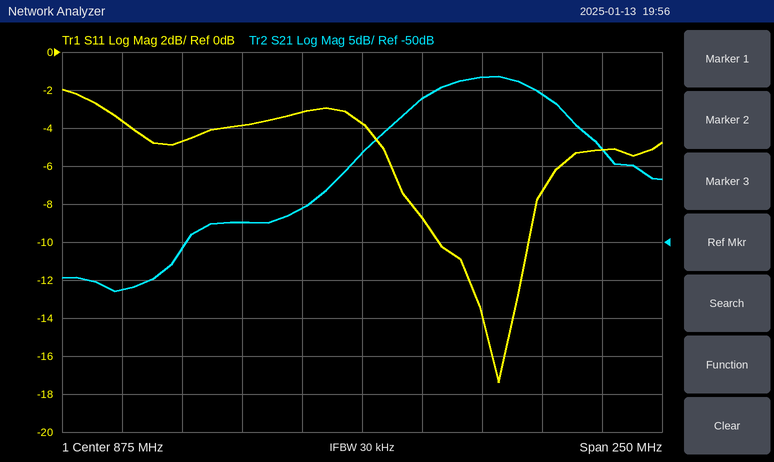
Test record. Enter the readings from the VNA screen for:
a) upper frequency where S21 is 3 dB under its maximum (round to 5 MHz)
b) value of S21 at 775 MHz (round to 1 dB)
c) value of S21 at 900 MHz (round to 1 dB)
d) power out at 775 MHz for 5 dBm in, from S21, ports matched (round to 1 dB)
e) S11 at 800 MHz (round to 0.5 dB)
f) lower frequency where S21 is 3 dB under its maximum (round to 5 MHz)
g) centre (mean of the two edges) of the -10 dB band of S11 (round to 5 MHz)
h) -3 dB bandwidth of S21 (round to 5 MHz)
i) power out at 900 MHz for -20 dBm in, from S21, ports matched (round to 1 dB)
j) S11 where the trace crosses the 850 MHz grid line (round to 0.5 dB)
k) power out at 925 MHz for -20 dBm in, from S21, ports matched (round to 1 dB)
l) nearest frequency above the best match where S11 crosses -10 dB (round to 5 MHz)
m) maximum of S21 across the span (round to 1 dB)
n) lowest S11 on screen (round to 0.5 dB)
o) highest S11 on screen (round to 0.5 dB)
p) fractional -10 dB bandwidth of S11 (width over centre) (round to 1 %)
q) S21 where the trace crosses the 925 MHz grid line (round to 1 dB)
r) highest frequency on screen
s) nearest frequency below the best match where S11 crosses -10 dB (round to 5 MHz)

955 MHz
-56 dB
-31 dB
-51 dBm
-4.5 dB
900 MHz
925 MHz
55 MHz
-51 dBm
-3.0 dB
-48 dBm
945 MHz
-28 dB
-17.5 dB
-2.0 dB
4 %
-28 dB
1 GHz
905 MHz
